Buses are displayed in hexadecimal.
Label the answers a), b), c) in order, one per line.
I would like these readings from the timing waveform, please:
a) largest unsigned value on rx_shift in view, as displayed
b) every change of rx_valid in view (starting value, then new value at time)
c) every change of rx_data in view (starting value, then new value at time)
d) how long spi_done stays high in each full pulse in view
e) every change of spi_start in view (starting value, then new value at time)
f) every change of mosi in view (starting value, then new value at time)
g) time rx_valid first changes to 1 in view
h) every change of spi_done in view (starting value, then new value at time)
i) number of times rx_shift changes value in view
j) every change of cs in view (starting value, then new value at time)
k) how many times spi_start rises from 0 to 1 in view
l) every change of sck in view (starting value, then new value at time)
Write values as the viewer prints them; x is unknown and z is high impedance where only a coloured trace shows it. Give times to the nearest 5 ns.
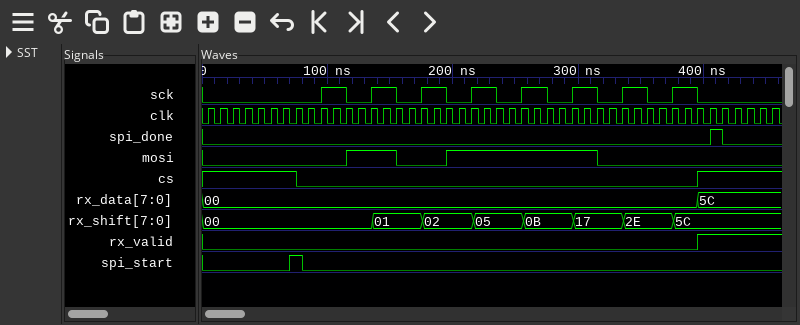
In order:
a) 5C
b) 0, 1 at 395 ns
c) 00, 5C at 395 ns
d) 10 ns
e) 0, 1 at 70 ns, 0 at 80 ns
f) 0, 1 at 115 ns, 0 at 155 ns, 1 at 195 ns, 0 at 315 ns
g) 395 ns
h) 0, 1 at 405 ns, 0 at 415 ns
i) 7
j) 1, 0 at 75 ns, 1 at 395 ns
k) 1
l) 0, 1 at 95 ns, 0 at 115 ns, 1 at 135 ns, 0 at 155 ns, 1 at 175 ns, 0 at 195 ns, 1 at 215 ns, 0 at 235 ns, 1 at 255 ns, 0 at 275 ns, 1 at 295 ns, 0 at 315 ns, 1 at 335 ns, 0 at 355 ns, 1 at 375 ns, 0 at 395 ns
